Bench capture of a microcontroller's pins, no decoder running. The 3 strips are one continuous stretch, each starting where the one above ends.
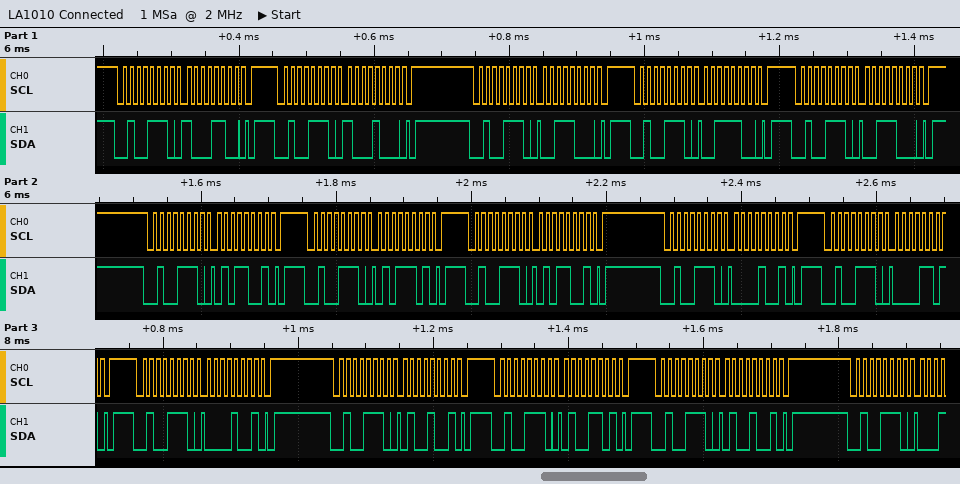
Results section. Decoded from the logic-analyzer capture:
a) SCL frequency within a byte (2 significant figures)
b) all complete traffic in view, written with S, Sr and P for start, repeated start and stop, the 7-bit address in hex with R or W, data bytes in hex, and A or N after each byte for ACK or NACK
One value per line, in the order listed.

100 kHz
S 27W A 8C A P S 27W A 88 A P S 27W A 38 A P S 27W A 3C A P S 27W A 38 A P S 27W A 59 A P S 27W A 5D A P S 27W A 59 A P S 27W A 09 A P S 27W A 0D A P S 27W A 09 A P S 27W A 49 A P S 27W A 4D A P S 27W A 49 A P S 27W A
